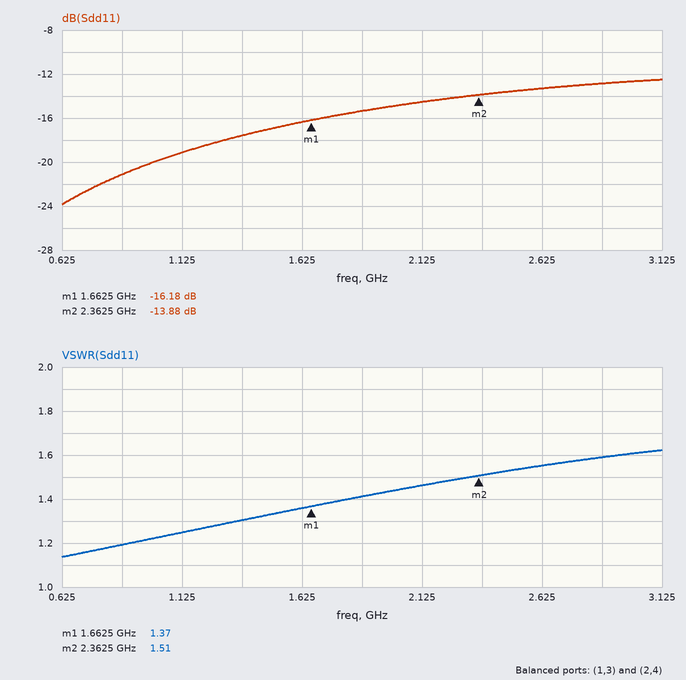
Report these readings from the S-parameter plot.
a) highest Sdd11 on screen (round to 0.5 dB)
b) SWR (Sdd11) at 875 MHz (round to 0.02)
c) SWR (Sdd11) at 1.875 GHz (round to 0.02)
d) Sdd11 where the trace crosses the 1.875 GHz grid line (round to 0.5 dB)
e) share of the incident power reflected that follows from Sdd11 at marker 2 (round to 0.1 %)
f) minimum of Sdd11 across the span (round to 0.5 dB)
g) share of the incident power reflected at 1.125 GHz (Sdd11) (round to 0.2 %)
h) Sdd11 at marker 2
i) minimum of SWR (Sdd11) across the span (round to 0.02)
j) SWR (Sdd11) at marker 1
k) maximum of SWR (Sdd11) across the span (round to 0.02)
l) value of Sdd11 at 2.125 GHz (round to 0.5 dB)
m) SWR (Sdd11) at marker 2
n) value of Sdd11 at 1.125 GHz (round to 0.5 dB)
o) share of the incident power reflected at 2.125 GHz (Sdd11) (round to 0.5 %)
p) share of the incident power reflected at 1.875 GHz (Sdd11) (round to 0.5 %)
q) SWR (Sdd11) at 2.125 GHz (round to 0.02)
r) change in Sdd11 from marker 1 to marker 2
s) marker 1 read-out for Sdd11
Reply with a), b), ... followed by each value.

a) -12.5 dB
b) 1.20
c) 1.42
d) -15.5 dB
e) 4.1 %
f) -24.0 dB
g) 1.2 %
h) -13.88 dB
i) 1.14
j) 1.37
k) 1.62
l) -14.5 dB
m) 1.51
n) -19.0 dB
o) 3.5 %
p) 3.0 %
q) 1.46
r) 2.30 dB
s) -16.18 dB
